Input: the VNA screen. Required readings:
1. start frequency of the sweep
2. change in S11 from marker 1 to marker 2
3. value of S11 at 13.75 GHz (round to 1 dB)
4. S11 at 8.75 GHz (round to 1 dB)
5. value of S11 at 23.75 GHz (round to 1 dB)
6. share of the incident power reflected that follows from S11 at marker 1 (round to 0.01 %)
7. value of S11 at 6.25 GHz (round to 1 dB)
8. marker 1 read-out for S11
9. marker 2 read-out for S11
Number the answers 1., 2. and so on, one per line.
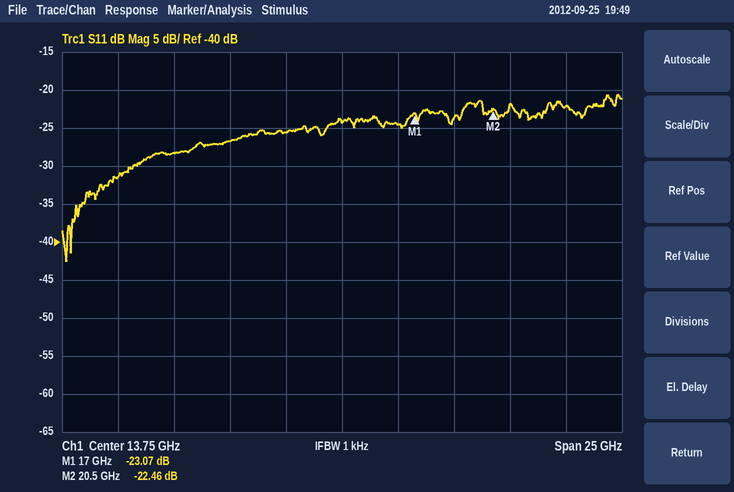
1. 1.25 GHz
2. 0.61 dB
3. -24 dB
4. -27 dB
5. -22 dB
6. 0.49 %
7. -28 dB
8. -23.07 dB
9. -22.46 dB
